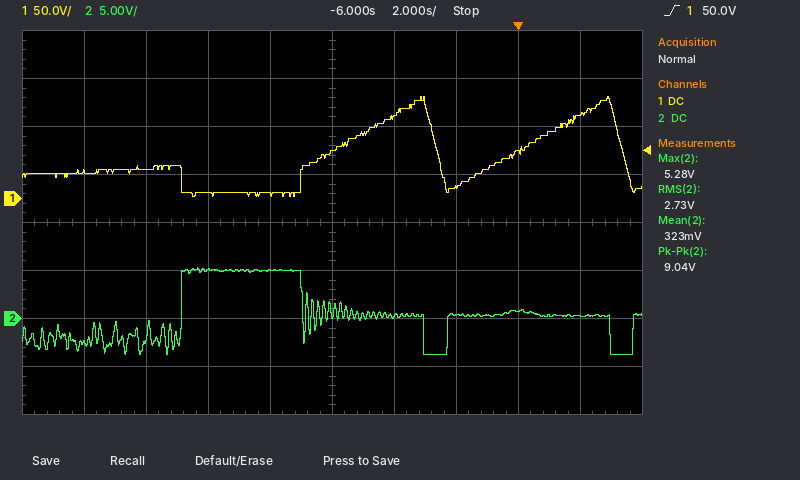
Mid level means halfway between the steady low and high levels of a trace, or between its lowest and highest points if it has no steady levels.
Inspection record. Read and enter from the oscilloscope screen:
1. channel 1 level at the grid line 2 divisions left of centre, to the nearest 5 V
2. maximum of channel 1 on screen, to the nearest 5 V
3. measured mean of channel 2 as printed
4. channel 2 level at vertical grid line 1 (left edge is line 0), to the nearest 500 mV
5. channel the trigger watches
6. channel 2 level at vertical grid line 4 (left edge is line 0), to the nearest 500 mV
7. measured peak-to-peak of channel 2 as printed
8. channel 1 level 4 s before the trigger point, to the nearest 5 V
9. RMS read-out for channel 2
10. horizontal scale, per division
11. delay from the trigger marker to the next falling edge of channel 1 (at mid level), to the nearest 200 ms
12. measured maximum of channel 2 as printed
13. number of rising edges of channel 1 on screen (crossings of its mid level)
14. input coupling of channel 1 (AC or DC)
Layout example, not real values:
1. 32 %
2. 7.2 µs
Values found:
1. 5 V
2. 105 V
3. 323 mV
4. -2.5 V
5. channel 1
6. 5.0 V
7. 9.04 V
8. 85 V
9. 2.73 V
10. 2 s
11. 3.4 s
12. 5.28 V
13. 2
14. DC
